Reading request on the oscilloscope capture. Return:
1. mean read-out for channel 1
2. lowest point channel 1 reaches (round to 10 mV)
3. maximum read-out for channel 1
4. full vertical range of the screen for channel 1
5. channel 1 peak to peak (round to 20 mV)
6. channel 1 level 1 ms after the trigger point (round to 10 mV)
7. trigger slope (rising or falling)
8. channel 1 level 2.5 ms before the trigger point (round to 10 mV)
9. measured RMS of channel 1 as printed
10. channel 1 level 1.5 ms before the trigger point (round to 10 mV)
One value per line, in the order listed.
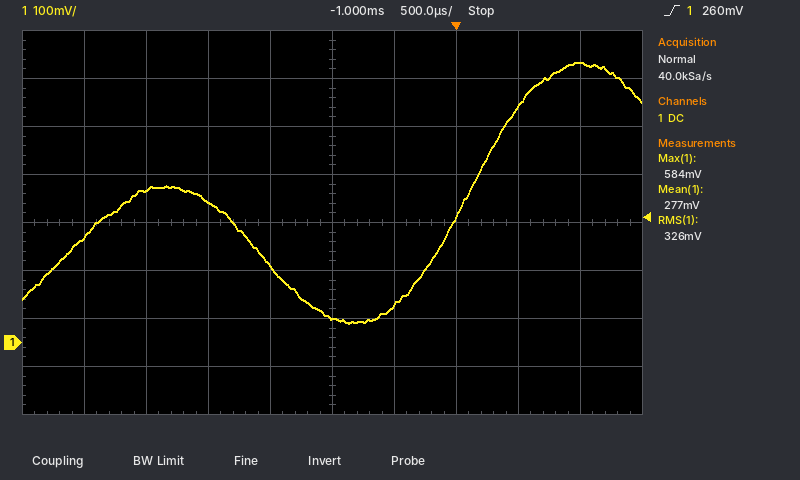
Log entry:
277 mV
40 mV
584 mV
800 mV
540 mV
580 mV
rising
320 mV
326 mV
160 mV
